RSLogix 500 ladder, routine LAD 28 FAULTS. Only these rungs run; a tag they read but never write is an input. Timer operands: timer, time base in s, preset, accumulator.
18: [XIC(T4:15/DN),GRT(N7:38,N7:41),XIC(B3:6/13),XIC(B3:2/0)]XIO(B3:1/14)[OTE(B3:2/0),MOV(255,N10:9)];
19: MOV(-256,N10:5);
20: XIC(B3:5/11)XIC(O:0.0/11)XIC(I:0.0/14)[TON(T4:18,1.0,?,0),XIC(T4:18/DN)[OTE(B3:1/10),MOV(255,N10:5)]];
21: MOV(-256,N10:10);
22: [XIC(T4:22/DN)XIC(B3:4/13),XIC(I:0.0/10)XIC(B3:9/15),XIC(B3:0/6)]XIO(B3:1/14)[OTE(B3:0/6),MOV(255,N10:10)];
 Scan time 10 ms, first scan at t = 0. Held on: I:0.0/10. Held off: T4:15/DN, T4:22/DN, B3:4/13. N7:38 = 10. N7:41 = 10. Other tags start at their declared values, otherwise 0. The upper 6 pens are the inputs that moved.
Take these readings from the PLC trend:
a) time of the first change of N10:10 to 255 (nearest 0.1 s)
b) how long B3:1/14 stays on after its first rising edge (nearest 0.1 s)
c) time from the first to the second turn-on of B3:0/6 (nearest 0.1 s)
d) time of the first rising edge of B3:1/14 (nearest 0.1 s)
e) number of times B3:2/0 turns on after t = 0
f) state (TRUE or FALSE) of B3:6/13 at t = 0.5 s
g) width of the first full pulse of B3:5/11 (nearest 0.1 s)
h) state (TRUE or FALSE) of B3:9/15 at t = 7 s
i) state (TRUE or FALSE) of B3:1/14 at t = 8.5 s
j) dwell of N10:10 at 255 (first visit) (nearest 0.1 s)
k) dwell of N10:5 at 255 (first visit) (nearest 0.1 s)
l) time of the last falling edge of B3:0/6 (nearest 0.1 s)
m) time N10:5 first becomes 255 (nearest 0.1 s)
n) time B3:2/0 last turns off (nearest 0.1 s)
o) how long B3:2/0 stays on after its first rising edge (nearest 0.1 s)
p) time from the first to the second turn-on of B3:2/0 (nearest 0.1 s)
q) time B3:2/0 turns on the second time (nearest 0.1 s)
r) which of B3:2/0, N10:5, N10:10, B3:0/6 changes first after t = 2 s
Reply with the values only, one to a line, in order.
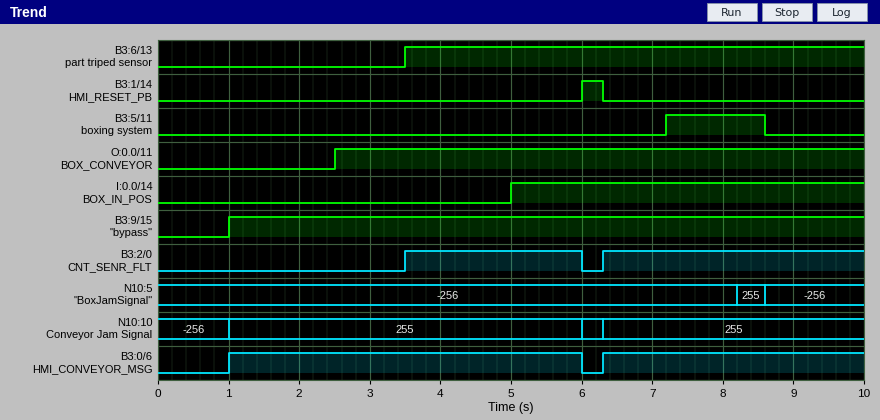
1.0 s
0.3 s
5.3 s
6.0 s
2
FALSE
1.4 s
TRUE
FALSE
5.0 s
0.4 s
6.0 s
8.2 s
6.0 s
2.5 s
2.8 s
6.3 s
B3:2/0
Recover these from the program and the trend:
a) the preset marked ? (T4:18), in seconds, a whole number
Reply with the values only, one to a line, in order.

1 s
